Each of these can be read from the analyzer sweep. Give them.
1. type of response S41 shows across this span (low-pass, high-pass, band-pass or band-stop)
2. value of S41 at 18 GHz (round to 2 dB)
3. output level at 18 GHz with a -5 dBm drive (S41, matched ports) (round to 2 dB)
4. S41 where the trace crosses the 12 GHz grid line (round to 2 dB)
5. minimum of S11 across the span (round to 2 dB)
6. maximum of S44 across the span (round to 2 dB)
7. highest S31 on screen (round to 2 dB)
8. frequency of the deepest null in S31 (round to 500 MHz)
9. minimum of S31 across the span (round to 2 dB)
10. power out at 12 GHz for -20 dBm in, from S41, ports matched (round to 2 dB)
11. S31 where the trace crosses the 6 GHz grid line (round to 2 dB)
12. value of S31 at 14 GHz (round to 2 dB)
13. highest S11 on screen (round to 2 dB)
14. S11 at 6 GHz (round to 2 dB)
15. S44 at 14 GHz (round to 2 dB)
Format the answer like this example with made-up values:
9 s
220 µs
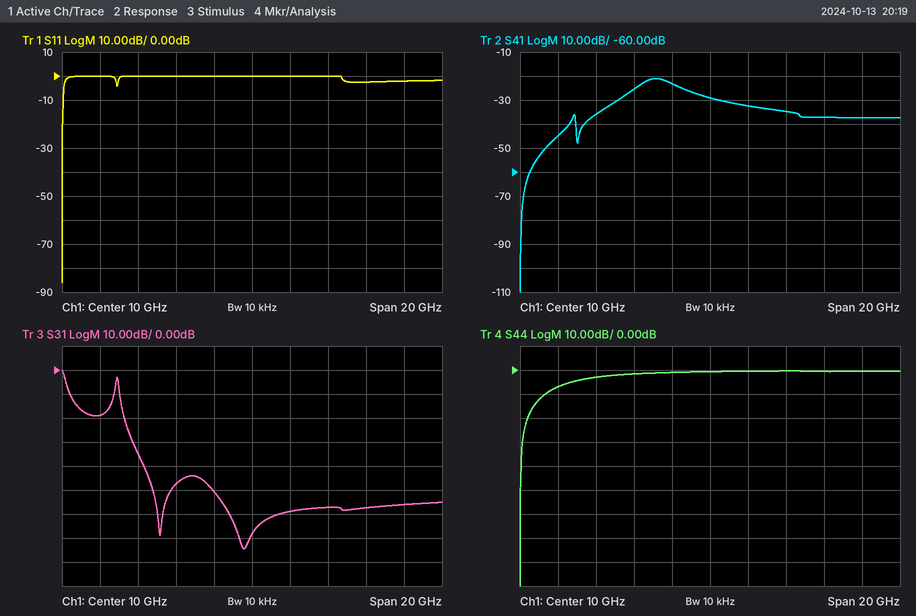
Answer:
band-pass
-38 dB
-42 dBm
-32 dB
-86 dB
0 dB
0 dB
9.5 GHz
-74 dB
-52 dBm
-48 dB
-58 dB
0 dB
0 dB
0 dB
